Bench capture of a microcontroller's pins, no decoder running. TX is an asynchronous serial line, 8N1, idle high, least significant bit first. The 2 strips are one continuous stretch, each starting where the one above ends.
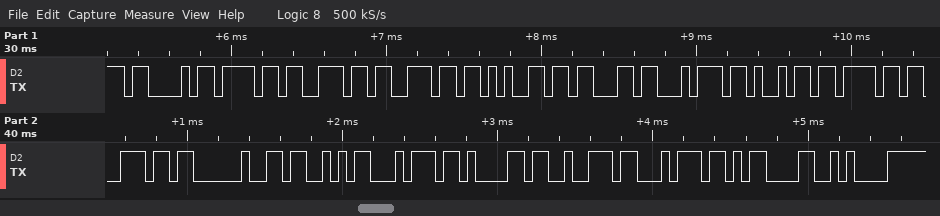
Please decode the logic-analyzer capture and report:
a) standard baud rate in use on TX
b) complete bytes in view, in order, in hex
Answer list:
19200 baud
43 6F 6E 6E 65 63 74 69 6F 6E 20 53 74 61 72 74 0D 0A
